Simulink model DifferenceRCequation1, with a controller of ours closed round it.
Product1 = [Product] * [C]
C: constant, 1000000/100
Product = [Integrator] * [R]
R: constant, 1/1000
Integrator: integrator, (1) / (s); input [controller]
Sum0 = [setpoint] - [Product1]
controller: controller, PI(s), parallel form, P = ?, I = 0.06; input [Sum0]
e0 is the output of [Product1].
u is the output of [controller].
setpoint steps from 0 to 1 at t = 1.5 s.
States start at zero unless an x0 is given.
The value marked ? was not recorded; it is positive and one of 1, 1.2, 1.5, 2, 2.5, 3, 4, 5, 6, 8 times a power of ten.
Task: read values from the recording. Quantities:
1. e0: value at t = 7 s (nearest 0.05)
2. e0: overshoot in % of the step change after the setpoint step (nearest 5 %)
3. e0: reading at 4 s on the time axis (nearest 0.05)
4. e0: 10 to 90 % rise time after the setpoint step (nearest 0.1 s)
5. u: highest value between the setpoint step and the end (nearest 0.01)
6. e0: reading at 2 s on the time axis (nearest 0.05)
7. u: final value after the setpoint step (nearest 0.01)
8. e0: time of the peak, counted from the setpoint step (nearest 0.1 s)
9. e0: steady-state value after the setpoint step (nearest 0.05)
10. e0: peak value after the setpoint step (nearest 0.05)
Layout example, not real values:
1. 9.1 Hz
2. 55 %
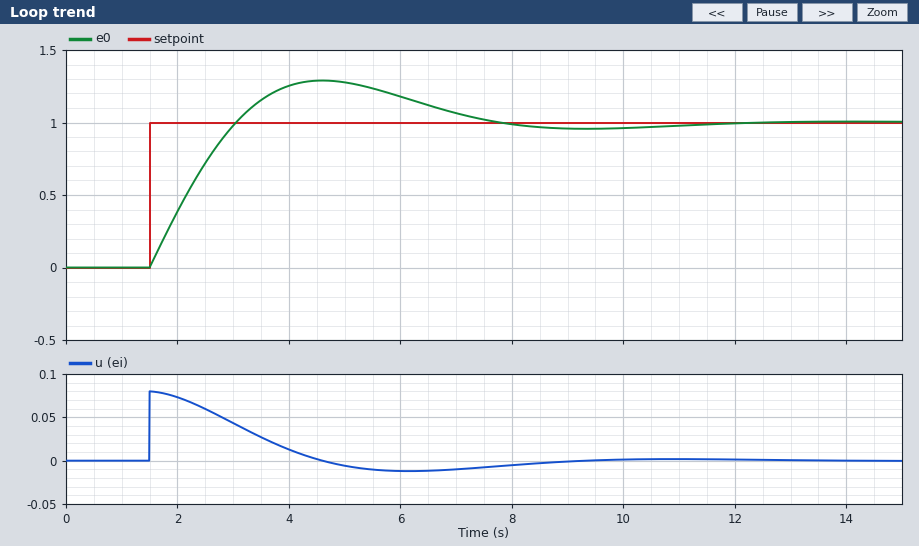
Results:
1. 1.05
2. 30 %
3. 1.25
4. 1.2 s
5. 0.08
6. 0.40
7. 0.00
8. 3.1 s
9. 1.00
10. 1.30
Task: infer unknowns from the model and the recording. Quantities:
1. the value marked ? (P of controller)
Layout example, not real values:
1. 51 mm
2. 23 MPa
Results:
1. 0.08
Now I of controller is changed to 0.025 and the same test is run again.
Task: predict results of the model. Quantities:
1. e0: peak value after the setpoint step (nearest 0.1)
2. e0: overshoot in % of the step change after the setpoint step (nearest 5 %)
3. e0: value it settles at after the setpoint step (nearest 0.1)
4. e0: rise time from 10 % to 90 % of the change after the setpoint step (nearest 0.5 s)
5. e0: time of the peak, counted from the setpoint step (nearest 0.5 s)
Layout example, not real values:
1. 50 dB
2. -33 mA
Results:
1. 1.2
2. 20 %
3. 1.0
4. 1.5 s
5. 4.5 s
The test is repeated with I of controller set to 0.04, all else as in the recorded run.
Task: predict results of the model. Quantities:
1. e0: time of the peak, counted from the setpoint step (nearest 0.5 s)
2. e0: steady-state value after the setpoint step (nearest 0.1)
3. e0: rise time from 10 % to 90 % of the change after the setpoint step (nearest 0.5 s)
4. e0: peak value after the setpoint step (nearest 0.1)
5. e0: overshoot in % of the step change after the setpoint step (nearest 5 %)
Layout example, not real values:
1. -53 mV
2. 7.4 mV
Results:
1. 3.5 s
2. 1.0
3. 1.5 s
4. 1.2
5. 25 %
